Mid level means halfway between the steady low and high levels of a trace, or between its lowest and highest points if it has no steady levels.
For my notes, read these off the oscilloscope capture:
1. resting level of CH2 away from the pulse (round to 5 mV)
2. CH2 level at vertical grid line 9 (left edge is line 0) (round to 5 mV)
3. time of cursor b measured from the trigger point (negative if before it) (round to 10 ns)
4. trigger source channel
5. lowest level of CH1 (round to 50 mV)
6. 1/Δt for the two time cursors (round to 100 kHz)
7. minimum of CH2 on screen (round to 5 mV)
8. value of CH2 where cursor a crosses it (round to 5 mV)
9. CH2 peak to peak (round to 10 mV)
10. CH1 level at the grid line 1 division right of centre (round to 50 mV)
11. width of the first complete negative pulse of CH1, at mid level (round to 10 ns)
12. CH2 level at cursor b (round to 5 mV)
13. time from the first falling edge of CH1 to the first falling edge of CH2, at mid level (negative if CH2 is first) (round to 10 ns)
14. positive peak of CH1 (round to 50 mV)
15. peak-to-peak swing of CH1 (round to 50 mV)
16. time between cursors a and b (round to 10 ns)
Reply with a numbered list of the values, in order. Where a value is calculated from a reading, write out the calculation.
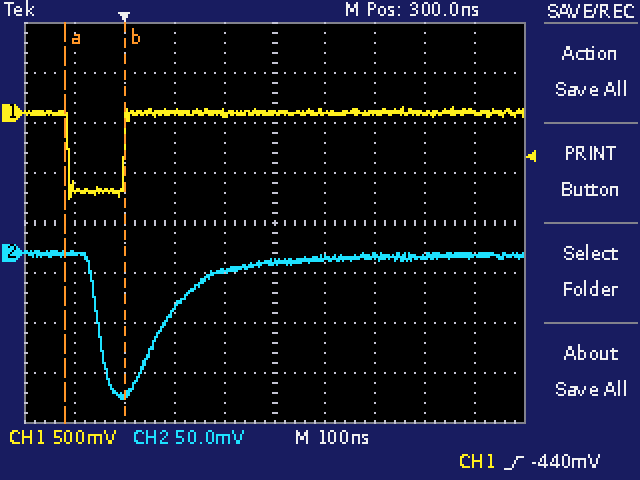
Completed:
1. -5 mV
2. 0 mV
3. 0 ns
4. CH1
5. -850 mV
6. 1 / 120 ns ≈ 8.3 MHz
7. -145 mV
8. 0 mV
9. 150 mV
10. 0 mV
11. 110 ns
12. -140 mV
13. +60 ns
14. 50 mV
15. 50 mV − (-850 mV) = 900 mV
16. 120 ns
